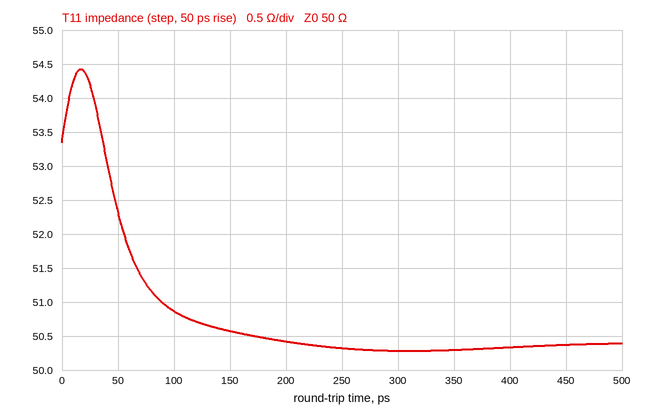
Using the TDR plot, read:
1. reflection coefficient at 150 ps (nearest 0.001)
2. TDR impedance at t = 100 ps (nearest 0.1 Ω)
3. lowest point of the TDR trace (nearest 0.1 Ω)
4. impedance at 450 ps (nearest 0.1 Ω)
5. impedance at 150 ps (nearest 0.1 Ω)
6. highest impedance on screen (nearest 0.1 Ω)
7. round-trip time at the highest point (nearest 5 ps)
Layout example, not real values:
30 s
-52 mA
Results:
+0.006
50.9 Ω
50.3 Ω
50.4 Ω
50.6 Ω
54.4 Ω
15 ps
